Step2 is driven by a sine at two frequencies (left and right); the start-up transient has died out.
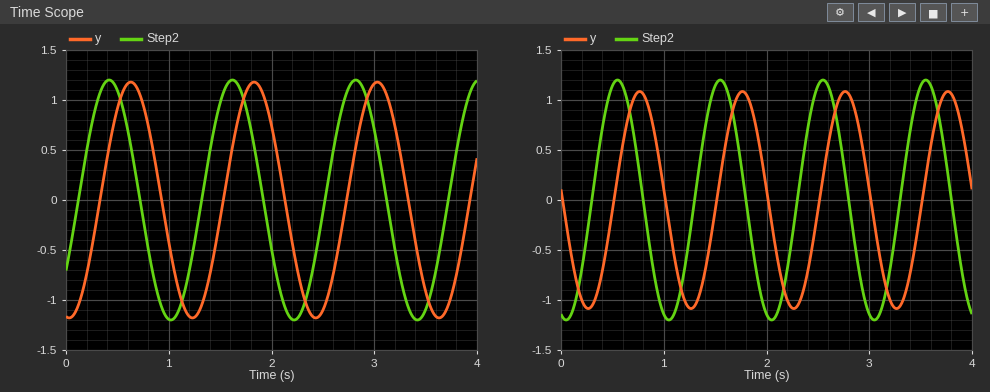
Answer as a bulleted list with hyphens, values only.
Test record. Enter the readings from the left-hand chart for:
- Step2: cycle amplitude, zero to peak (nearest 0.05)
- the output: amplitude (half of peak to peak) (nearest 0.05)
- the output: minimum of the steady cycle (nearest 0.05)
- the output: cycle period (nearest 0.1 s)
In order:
- 1.20
- 1.20
- -1.20
- 1.2 s
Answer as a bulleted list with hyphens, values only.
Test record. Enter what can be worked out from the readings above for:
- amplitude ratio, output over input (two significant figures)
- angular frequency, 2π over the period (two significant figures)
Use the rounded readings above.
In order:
- 1.0
- 5.2 rad/s
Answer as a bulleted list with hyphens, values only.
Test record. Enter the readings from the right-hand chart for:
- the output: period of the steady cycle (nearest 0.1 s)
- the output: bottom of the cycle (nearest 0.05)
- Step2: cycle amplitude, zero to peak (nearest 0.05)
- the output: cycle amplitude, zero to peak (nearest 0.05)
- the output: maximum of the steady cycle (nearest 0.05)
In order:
- 1.0 s
- -1.10
- 1.20
- 1.10
- 1.10
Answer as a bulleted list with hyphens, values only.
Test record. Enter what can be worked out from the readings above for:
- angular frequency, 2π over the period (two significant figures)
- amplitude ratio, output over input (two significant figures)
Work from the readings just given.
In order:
- 6.3 rad/s
- 0.92
